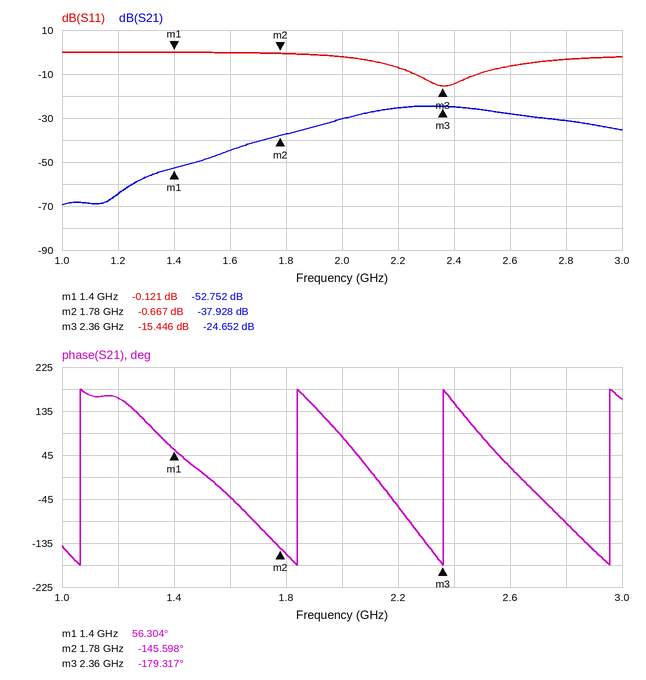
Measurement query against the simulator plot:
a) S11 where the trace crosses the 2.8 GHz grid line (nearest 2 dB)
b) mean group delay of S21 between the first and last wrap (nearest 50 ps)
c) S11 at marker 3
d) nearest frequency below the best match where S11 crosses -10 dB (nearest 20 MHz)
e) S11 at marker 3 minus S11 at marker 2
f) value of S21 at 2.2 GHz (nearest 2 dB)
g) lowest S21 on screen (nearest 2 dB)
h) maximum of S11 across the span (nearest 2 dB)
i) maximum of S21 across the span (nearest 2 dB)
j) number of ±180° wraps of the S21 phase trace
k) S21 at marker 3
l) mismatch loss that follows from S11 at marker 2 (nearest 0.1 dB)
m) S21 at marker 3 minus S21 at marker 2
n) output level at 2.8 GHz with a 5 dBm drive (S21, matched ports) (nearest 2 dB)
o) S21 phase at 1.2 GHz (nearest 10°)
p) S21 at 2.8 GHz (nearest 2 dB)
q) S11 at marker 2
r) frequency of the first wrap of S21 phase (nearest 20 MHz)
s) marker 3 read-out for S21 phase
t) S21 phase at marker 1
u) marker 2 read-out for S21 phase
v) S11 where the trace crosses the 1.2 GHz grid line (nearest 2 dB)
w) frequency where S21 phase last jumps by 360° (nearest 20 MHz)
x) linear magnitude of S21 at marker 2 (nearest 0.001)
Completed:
-4 dB
1.60 ns
-15.446 dB
2.26 GHz
-14.779 dB
-26 dB
-70 dB
0 dB
-24 dB
4
-24.652 dB
8.5 dB
13.276 dB
-26 dBm
160°
-32 dB
-0.667 dB
1.06 GHz
-179.317°
56.304°
-145.598°
0 dB
2.96 GHz
0.013
